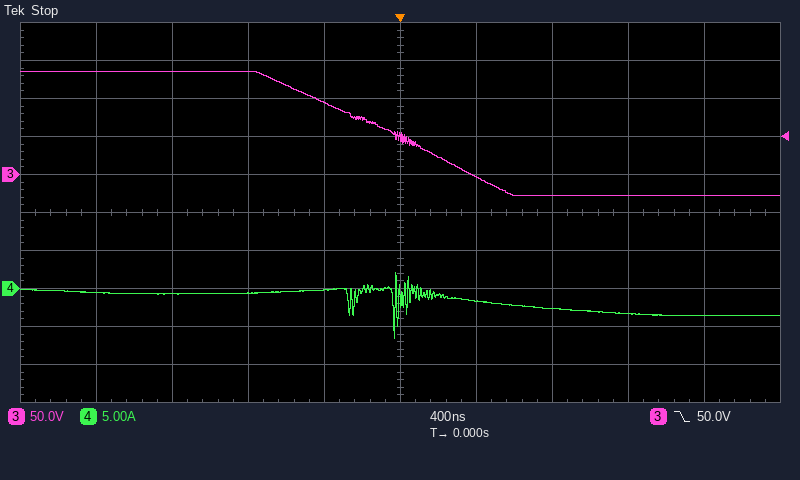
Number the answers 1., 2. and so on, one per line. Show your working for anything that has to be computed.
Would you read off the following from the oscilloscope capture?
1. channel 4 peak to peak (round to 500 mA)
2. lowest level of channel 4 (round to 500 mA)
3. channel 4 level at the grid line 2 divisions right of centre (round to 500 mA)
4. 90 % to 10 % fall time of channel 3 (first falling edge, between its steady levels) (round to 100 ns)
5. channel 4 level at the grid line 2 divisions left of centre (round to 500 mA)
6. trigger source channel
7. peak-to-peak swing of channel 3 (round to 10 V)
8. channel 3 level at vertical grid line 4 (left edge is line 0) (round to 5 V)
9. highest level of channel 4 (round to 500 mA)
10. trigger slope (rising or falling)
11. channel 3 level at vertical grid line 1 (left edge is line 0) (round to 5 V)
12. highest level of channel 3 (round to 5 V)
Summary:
1. 2.0 A − (-6.5 A) = 8.5 A
2. -6.5 A
3. -2.5 A
4. 1.1 µs
5. -500 mA
6. channel 3
7. 160 V
8. 95 V
9. 2.0 A
10. falling
11. 135 V
12. 135 V
